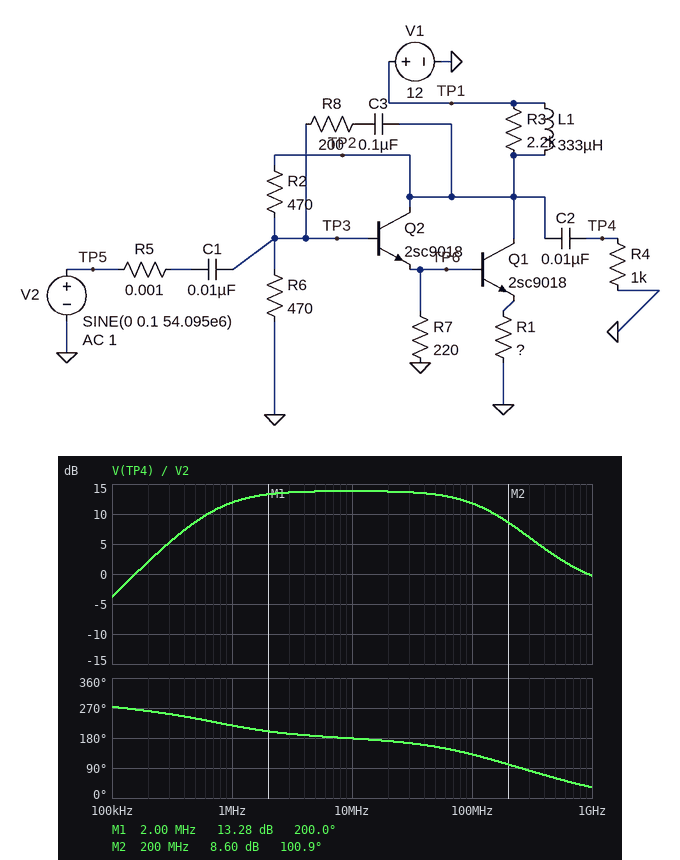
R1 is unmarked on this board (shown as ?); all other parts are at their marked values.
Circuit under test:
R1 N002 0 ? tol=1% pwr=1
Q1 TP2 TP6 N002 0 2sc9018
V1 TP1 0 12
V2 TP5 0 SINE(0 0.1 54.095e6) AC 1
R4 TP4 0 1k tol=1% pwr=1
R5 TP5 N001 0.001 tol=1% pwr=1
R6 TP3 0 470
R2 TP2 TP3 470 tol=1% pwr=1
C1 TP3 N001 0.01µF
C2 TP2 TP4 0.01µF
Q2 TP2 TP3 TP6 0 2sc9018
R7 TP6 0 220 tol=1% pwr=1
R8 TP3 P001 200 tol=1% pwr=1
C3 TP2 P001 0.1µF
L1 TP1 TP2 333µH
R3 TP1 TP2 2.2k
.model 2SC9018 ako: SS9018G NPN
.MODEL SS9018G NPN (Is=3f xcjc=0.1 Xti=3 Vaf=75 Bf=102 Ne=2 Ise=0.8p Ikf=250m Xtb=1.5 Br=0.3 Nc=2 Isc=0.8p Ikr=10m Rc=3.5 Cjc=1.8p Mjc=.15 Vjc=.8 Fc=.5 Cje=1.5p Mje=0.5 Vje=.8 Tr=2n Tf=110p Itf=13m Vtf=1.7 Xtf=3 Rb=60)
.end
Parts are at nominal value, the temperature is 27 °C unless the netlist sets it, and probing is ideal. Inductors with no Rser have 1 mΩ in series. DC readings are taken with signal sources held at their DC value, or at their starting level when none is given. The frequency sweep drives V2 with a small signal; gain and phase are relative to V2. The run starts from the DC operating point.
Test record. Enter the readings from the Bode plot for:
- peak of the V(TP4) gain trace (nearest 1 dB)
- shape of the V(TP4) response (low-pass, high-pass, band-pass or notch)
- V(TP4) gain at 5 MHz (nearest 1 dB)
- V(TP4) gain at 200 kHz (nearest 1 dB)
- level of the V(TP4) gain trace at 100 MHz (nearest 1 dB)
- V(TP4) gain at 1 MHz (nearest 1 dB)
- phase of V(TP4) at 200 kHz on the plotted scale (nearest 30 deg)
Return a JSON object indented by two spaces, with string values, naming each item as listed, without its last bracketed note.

{
  "peak of the V(TP4) gain trace": "14 dB",
  "shape of the V(TP4) response": "band-pass",
  "V(TP4) gain at 5 MHz": "14 dB",
  "V(TP4) gain at 200 kHz": "2 dB",
  "level of the V(TP4) gain trace at 100 MHz": "12 dB",
  "V(TP4) gain at 1 MHz": "12 dB",
  "phase of V(TP4) at 200 kHz on the plotted scale": "270 deg"
}
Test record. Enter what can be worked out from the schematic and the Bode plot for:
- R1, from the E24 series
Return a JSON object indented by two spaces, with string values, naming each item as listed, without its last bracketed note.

{
  "R1, from the E24 series": "20 Ω"
}
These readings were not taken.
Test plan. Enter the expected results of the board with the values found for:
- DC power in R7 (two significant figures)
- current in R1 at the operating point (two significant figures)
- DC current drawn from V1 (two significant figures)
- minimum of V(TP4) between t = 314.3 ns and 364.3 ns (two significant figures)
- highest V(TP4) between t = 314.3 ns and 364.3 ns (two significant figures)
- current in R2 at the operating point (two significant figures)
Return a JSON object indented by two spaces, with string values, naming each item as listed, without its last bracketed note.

{
  "DC power in R7": "120 mW",
  "current in R1 at the operating point": "210 mA",
  "DC current drawn from V1": "240 mA",
  "minimum of V(TP4) between t = 314.3 ns and 364.3 ns": "-440 mV",
  "highest V(TP4) between t = 314.3 ns and 364.3 ns": "460 mV",
  "current in R2 at the operating point": "13 mA"
}
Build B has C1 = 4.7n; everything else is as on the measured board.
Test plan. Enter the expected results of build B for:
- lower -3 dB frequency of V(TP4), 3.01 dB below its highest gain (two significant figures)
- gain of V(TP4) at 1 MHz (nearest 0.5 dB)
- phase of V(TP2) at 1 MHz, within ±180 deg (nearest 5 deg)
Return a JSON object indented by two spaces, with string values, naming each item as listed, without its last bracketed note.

{
  "lower -3 dB frequency of V(TP4), 3.01 dB below its highest gain": "1.5 MHz",
  "gain of V(TP4) at 1 MHz": "8.5 dB",
  "phase of V(TP2) at 1 MHz, within ±180 deg": "-125 deg"
}
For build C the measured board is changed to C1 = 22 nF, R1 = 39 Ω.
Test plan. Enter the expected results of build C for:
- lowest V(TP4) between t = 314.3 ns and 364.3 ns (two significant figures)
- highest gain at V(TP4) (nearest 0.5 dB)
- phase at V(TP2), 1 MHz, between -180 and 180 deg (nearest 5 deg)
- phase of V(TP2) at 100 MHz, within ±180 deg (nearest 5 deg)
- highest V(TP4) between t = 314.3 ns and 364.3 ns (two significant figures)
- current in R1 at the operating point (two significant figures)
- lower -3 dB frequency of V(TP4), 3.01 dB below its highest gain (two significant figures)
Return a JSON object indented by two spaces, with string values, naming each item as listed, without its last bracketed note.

{
  "lowest V(TP4) between t = 314.3 ns and 364.3 ns": "-250 mV",
  "highest gain at V(TP4)": "8.0 dB",
  "phase at V(TP2), 1 MHz, between -180 and 180 deg": "-165 deg",
  "phase of V(TP2) at 100 MHz, within ±180 deg": "150 deg",
  "highest V(TP4) between t = 314.3 ns and 364.3 ns": "250 mV",
  "current in R1 at the operating point": "110 mA",
  "lower -3 dB frequency of V(TP4), 3.01 dB below its highest gain": "240 kHz"
}
